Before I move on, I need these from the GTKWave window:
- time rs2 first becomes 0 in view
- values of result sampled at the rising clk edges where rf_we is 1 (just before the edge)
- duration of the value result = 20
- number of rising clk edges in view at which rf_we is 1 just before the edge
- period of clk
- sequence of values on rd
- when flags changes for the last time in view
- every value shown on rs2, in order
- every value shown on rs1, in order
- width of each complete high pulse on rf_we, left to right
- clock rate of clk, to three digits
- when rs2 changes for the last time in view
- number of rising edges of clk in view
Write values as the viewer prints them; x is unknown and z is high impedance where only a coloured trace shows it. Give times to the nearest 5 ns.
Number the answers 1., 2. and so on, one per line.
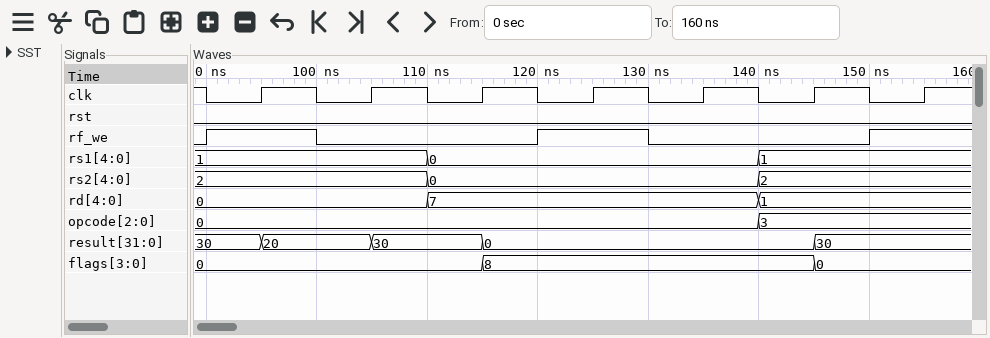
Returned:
1. 110 ns
2. 30, 0, 30
3. 10 ns
4. 3
5. 10 ns
6. 0, 7, 1
7. 145 ns
8. 2, 0, 2
9. 1, 0, 1
10. 10 ns, 10 ns
11. 100 MHz
12. 140 ns
13. 7
